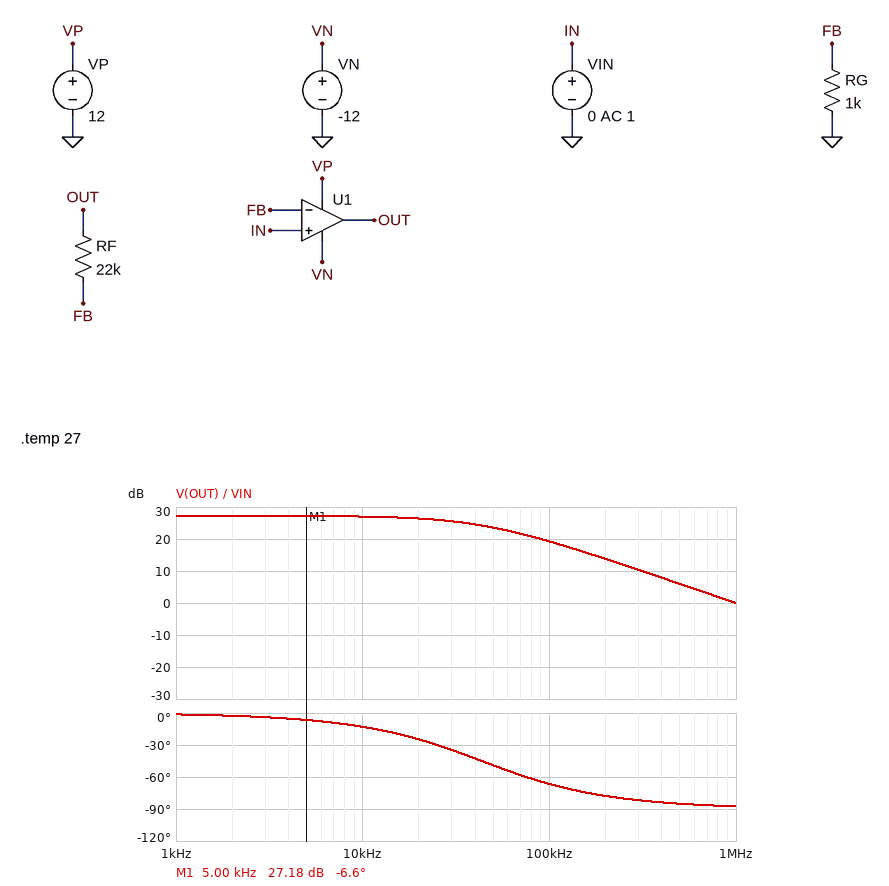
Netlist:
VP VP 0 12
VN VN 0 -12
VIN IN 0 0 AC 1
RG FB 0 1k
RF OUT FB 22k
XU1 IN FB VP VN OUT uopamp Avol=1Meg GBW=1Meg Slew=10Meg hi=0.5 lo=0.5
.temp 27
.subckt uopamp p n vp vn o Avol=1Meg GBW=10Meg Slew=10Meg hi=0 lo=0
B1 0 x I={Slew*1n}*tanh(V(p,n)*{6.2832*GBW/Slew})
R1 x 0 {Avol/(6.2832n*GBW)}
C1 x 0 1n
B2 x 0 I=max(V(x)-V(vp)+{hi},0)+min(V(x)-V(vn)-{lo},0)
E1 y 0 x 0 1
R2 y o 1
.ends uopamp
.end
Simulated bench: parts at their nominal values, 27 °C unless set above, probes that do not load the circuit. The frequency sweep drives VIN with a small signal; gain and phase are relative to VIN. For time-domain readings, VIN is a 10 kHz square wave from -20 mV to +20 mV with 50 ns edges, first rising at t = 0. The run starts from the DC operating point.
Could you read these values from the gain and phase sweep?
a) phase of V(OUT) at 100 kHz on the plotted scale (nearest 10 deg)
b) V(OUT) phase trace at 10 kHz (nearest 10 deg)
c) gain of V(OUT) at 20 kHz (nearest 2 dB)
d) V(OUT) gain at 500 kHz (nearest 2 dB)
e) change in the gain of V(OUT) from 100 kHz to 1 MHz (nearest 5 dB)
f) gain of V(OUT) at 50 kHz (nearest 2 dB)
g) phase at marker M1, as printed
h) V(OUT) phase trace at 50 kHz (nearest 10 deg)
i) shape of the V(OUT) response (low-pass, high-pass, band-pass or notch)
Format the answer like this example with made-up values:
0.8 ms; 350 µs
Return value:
-70 deg; -10 deg; 26 dB; 6 dB; -20 dB; 24 dB; -6.6 deg; -50 deg; low-pass
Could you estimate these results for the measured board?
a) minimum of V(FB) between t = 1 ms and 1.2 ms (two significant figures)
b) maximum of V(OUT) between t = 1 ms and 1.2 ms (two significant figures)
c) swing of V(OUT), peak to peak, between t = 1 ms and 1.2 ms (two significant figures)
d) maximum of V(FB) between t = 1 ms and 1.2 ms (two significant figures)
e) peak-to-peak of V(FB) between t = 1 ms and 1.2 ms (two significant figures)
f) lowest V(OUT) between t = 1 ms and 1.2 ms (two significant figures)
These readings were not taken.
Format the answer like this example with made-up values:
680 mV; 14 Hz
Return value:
-20 mV; 460 mV; 920 mV; 20 mV; 40 mV; -460 mV
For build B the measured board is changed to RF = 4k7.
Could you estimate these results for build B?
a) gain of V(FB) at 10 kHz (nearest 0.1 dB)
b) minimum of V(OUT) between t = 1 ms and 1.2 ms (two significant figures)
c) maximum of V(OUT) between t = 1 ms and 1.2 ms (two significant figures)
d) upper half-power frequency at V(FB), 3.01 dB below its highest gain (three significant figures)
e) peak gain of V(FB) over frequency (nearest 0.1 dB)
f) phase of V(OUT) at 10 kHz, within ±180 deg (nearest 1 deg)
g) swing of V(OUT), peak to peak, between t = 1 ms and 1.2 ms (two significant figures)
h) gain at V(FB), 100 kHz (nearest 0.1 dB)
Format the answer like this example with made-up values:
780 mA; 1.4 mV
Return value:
0 dB; -110 mV; 110 mV; 175 kHz; 0 dB; -3 deg; 230 mV; -1.2 dB
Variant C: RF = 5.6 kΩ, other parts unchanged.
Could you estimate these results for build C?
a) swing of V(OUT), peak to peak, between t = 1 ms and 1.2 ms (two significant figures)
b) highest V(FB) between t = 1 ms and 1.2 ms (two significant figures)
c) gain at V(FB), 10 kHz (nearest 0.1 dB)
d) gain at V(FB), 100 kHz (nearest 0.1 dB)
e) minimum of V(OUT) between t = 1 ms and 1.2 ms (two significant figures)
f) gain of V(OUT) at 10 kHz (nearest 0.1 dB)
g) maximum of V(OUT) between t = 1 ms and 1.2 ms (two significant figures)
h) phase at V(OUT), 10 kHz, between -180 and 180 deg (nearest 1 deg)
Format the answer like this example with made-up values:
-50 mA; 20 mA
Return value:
260 mV; 20 mV; 0 dB; -1.6 dB; -130 mV; 16.4 dB; 130 mV; -4 deg
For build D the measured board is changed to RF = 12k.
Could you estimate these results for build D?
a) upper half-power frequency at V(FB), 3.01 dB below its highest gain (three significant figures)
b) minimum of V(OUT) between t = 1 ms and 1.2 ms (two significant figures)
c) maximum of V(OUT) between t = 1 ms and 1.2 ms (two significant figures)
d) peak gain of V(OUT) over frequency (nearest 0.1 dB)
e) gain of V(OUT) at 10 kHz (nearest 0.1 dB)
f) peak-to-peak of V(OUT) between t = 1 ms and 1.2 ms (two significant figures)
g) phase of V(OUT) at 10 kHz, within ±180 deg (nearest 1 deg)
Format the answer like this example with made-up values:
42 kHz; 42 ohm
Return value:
76.9 kHz; -260 mV; 260 mV; 22.3 dB; 22.2 dB; 520 mV; -7 deg
